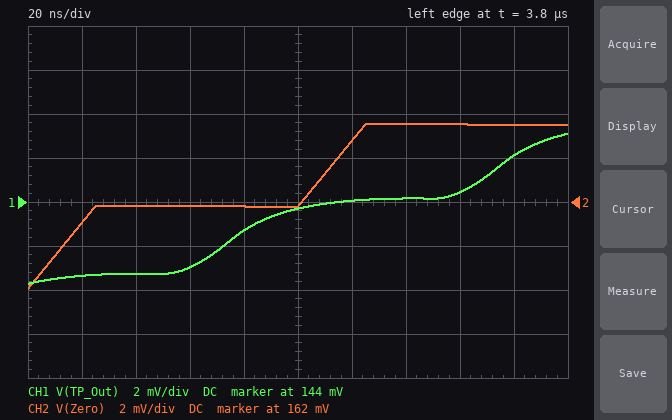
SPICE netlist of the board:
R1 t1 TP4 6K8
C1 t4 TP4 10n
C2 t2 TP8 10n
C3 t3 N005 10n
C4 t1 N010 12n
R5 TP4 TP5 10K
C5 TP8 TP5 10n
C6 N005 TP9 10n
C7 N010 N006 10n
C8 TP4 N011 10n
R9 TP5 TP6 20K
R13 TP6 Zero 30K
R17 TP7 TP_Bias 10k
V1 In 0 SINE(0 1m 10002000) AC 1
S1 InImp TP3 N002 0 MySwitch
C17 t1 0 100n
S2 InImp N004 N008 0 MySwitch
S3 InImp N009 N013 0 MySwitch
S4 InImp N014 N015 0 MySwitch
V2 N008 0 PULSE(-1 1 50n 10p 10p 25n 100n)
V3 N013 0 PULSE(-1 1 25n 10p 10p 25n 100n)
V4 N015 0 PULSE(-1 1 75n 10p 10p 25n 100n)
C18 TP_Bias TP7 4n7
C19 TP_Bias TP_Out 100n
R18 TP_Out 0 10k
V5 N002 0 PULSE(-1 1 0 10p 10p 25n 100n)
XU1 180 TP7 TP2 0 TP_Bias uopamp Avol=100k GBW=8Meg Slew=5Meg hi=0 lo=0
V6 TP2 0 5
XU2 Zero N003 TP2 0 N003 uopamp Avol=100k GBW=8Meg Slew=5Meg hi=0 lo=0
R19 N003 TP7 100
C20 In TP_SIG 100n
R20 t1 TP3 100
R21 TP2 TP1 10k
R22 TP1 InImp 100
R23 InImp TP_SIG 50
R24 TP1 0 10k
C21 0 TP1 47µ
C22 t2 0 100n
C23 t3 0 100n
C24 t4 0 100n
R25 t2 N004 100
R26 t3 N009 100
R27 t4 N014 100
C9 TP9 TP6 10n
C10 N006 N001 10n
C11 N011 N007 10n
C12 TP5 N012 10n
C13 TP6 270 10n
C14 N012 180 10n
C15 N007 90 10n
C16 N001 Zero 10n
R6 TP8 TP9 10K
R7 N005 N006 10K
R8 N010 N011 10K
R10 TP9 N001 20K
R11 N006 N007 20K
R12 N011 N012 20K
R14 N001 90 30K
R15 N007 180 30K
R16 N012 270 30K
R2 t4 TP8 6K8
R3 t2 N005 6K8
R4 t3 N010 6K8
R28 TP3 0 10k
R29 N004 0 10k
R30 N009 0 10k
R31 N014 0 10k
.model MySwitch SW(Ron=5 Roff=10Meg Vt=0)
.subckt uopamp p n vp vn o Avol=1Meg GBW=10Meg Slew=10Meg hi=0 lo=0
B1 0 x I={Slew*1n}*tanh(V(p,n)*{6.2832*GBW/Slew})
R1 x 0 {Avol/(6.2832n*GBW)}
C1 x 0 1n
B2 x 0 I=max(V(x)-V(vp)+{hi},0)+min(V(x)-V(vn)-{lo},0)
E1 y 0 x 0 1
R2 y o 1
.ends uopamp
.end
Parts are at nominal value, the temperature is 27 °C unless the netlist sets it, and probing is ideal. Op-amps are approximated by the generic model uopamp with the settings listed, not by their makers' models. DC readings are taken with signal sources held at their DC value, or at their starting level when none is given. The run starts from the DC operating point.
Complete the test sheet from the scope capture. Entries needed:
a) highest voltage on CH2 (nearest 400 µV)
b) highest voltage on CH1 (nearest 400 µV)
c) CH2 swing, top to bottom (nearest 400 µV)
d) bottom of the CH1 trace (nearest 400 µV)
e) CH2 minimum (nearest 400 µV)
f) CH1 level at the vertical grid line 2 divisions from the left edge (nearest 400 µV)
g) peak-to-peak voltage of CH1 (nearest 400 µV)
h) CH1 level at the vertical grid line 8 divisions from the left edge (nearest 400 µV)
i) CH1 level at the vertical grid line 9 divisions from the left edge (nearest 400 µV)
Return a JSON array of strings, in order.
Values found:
["165.6 mV", "147.2 mV", "7.6 mV", "140.4 mV", "158.0 mV", "140.8 mV", "6.8 mV", "144.4 mV", "146.0 mV"]
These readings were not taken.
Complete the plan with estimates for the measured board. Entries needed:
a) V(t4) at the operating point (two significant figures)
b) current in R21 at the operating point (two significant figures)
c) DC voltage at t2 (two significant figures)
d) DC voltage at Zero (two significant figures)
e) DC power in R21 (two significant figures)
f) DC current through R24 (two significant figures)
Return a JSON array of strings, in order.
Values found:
["2.5 mV", "250 µA", "2.5 mV", "2.5 mV", "630 µW", "250 µA"]
